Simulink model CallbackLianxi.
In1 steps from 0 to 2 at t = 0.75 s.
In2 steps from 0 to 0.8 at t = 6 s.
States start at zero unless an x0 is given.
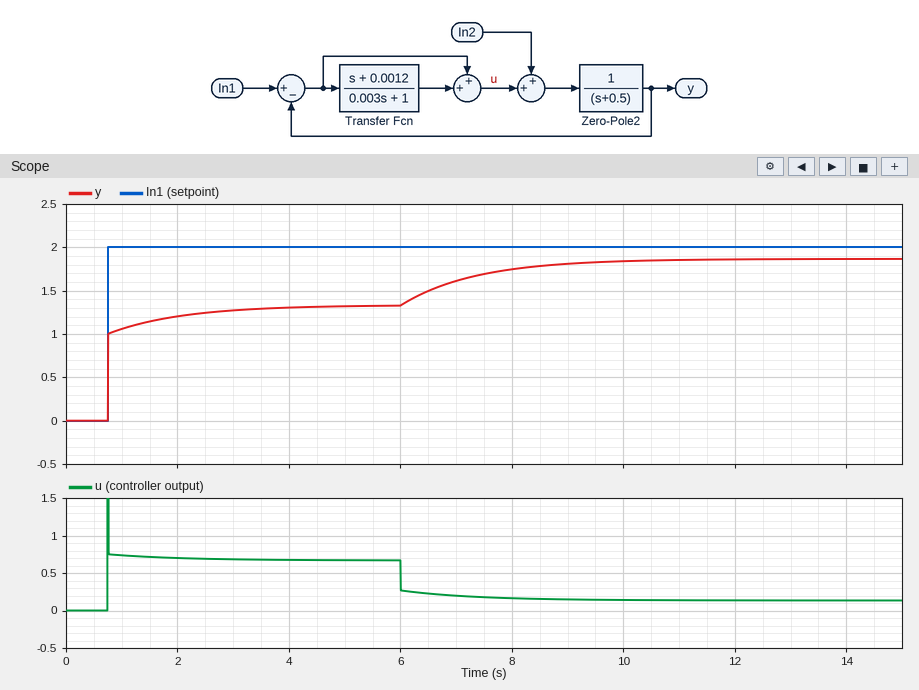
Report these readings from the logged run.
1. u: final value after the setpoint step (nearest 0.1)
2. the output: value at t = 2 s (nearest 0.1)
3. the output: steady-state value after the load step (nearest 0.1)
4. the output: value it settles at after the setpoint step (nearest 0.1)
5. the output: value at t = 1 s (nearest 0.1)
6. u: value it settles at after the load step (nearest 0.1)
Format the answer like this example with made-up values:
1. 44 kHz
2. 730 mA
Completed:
1. 0.7
2. 1.2
3. 1.9
4. 1.3
5. 1.1
6. 0.1
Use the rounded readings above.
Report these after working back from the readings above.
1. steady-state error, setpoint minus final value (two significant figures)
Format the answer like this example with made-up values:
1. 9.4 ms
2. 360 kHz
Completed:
1. 0.70
